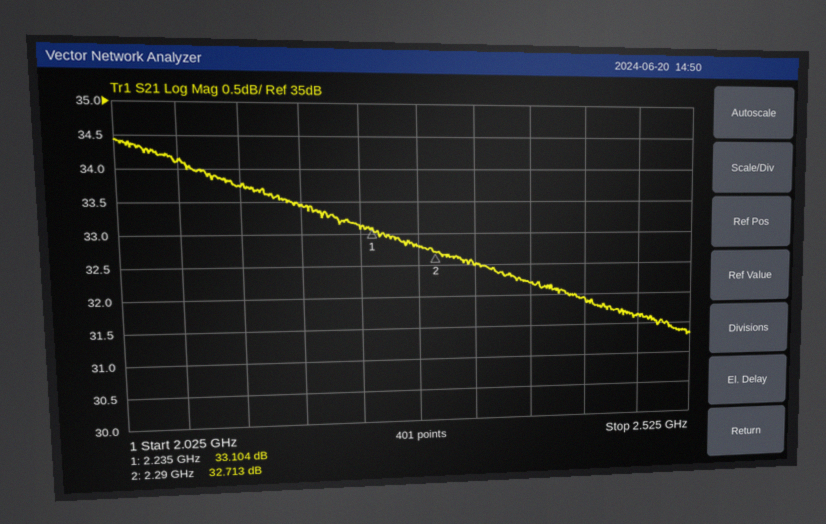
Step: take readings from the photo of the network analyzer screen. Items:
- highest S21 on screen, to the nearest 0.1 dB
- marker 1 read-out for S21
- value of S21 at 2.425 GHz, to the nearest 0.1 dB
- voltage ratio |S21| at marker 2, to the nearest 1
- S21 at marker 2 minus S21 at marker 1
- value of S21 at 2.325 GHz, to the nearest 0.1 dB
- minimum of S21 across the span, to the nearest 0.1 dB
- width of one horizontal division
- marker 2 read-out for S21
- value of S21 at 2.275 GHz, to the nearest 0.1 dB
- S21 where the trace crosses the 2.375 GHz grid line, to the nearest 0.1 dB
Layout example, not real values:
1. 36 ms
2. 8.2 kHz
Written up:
1. 34.4 dB
2. 33.104 dB
3. 31.9 dB
4. 43
5. -0.391 dB
6. 32.5 dB
7. 31.3 dB
8. 50 MHz
9. 32.713 dB
10. 32.8 dB
11. 32.2 dB
